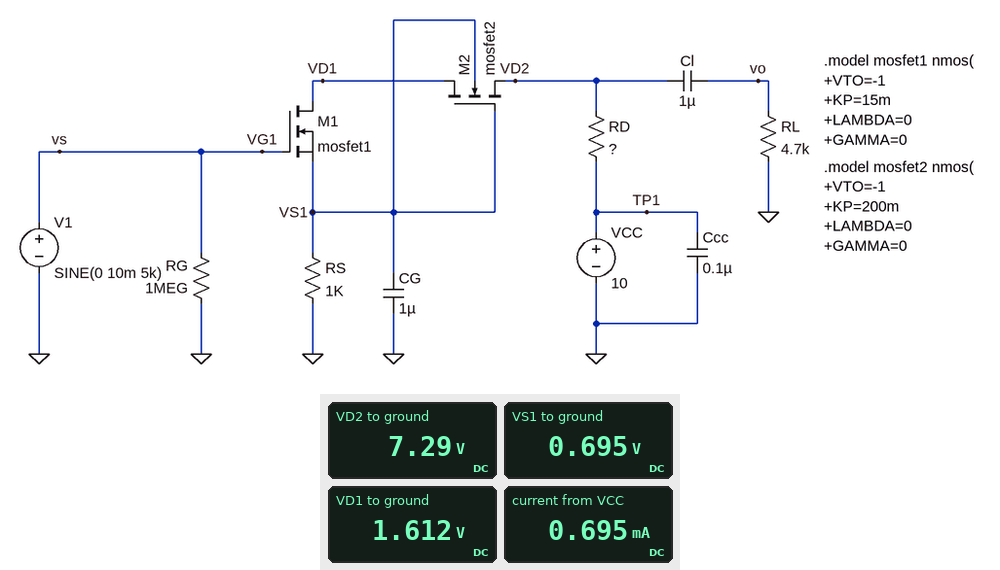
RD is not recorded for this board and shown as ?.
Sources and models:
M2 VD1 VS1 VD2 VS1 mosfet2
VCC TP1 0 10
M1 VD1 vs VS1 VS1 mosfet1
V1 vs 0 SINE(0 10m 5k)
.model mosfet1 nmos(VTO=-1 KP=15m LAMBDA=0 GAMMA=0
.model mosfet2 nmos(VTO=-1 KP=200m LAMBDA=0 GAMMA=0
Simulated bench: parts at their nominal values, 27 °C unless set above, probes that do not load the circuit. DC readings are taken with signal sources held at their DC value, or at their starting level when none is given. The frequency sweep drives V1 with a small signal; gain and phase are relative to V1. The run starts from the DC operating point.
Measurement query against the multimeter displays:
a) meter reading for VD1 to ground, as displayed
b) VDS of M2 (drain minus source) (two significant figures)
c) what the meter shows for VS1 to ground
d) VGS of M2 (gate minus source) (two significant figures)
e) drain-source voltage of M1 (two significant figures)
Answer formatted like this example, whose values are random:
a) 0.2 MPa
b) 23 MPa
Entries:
a) 1.612 V
b) -5.7 V
c) 0.695 V
d) -6.6 V
e) 920 mV
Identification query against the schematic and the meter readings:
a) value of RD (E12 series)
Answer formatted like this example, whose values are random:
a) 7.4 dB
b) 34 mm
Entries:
a) 3.9 kΩ
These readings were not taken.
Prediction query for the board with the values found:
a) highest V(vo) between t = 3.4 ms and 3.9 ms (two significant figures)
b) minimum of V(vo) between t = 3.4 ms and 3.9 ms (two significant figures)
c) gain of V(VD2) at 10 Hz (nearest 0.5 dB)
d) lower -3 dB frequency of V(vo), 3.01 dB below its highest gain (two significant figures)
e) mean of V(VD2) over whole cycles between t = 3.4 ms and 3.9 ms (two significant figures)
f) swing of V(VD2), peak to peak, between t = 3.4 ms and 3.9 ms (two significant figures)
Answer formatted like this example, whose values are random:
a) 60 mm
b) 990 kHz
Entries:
a) 95 mV
b) -97 mV
c) 9.5 dB
d) 860 Hz
e) 7.3 V
f) 190 mV
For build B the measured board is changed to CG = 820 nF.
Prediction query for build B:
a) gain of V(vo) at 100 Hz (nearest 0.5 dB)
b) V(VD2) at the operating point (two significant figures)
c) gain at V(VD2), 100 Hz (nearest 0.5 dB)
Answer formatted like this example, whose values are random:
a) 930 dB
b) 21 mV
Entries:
a) 5.5 dB
b) 7.3 V
c) 6.0 dB
